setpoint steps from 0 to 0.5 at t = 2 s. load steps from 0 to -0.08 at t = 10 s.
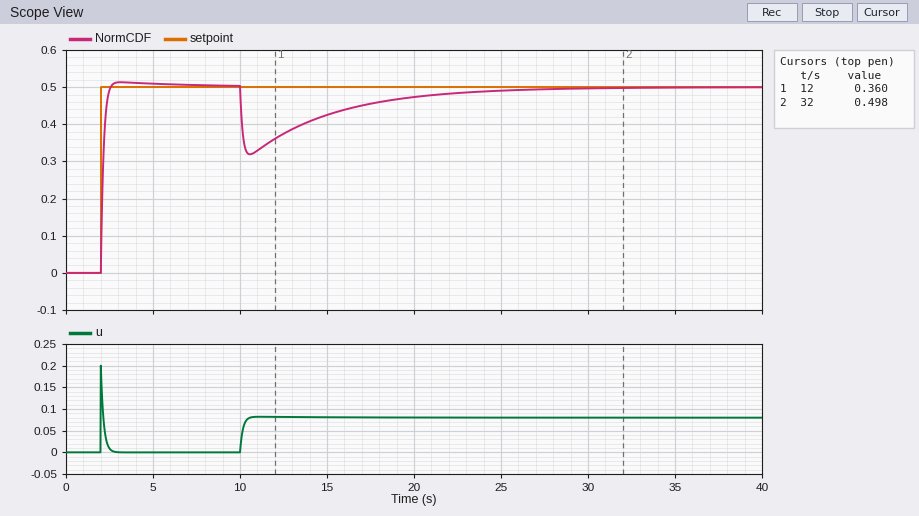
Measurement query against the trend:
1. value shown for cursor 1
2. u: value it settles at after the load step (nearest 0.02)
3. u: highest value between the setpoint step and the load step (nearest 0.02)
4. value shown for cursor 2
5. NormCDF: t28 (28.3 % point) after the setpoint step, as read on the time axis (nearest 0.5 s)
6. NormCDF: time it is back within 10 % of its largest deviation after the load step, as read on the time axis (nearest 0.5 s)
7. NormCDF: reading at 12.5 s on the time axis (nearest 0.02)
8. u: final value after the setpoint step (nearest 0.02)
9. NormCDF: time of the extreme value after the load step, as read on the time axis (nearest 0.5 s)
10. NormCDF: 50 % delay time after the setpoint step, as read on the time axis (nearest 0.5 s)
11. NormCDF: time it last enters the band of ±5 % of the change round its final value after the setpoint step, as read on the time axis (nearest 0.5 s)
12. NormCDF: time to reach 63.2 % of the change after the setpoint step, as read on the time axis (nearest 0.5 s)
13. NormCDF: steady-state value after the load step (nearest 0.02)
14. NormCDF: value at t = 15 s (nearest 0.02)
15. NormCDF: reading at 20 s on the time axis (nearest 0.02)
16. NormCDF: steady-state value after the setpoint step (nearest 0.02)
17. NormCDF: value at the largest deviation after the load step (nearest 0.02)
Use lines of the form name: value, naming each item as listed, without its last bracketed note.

value shown for cursor 1: 0.360
u: value it settles at after the load step: 0.08
u: highest value between the setpoint step and the load step: 0.20
value shown for cursor 2: 0.498
NormCDF: t28 (28.3 % point) after the setpoint step, as read on the time axis: 2.0 s
NormCDF: time it is back within 10 % of its largest deviation after the load step, as read on the time axis: 22.0 s
NormCDF: reading at 12.5 s on the time axis: 0.38
u: final value after the setpoint step: 0.00
NormCDF: time of the extreme value after the load step, as read on the time axis: 10.5 s
NormCDF: 50 % delay time after the setpoint step, as read on the time axis: 2.0 s
NormCDF: time it last enters the band of ±5 % of the change round its final value after the setpoint step, as read on the time axis: 2.5 s
NormCDF: time to reach 63.2 % of the change after the setpoint step, as read on the time axis: 2.0 s
NormCDF: steady-state value after the load step: 0.50
NormCDF: value at t = 15 s: 0.42
NormCDF: reading at 20 s on the time axis: 0.48
NormCDF: steady-state value after the setpoint step: 0.50
NormCDF: value at the largest deviation after the load step: 0.32
